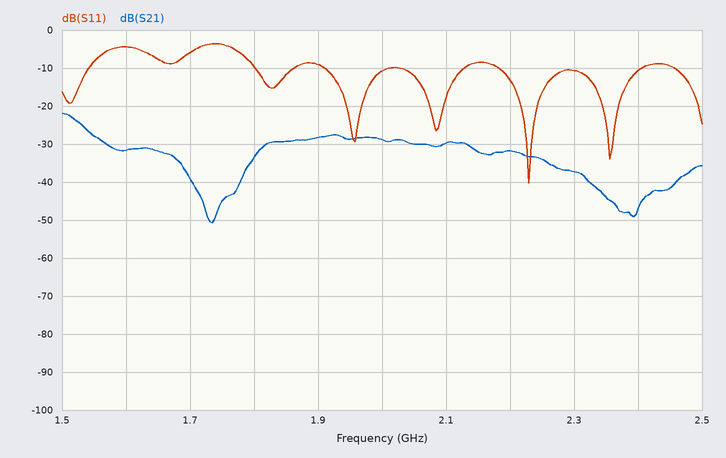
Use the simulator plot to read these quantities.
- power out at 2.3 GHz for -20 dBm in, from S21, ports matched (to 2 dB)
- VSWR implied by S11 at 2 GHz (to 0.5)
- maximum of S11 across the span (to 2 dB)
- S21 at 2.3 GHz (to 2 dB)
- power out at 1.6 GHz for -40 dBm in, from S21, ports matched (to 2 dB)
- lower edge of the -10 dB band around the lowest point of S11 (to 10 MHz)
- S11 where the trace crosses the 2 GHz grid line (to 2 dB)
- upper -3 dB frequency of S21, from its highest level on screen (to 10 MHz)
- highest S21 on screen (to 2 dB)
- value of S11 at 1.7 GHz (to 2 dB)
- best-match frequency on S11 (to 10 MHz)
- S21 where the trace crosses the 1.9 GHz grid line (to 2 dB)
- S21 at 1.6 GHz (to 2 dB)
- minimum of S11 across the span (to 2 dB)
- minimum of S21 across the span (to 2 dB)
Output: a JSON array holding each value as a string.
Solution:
["-58 dBm", "2.0", "-4 dB", "-38 dB", "-72 dBm", "2.18 GHz", "-10 dB", "1.53 GHz", "-22 dB", "-6 dB", "2.23 GHz", "-28 dB", "-32 dB", "-40 dB", "-50 dB"]
